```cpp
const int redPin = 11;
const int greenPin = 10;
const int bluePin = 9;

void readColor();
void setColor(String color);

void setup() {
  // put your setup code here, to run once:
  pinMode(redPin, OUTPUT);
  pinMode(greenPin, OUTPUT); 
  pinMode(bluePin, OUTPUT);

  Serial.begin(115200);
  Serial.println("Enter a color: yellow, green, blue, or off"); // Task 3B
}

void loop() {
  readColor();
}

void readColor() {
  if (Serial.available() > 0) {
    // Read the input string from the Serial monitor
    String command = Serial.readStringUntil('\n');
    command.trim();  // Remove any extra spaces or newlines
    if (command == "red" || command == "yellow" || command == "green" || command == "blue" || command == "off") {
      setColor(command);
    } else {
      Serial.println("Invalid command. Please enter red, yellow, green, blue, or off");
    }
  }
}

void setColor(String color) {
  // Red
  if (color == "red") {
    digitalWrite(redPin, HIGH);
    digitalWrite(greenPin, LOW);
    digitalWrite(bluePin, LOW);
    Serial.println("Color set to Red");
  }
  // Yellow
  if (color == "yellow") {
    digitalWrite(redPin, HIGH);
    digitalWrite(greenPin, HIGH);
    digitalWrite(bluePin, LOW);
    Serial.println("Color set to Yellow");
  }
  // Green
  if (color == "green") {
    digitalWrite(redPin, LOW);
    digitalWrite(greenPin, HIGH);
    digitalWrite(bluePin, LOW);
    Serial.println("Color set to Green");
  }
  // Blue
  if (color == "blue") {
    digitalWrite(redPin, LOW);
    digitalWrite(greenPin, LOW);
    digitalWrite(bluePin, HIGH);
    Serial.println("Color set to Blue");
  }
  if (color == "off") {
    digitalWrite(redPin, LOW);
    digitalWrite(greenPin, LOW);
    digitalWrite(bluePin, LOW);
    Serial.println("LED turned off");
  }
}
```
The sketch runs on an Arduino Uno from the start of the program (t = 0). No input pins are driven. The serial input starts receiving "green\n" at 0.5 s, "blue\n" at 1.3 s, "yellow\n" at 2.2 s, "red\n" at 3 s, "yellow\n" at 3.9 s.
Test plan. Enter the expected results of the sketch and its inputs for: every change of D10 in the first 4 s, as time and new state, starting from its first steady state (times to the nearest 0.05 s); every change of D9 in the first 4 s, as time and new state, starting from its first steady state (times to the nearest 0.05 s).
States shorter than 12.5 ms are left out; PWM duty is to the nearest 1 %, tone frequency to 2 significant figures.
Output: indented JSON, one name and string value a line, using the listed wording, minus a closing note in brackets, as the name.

{
  "every change of D10 in the first 4 s, as time and new state, starting from its first steady state": "0 s low; 0.5 s high; 1.3 s low; 2.2 s high; 3 s low; 3.9 s high",
  "every change of D9 in the first 4 s, as time and new state, starting from its first steady state": "0 s low; 1.3 s high; 2.2 s low"
}
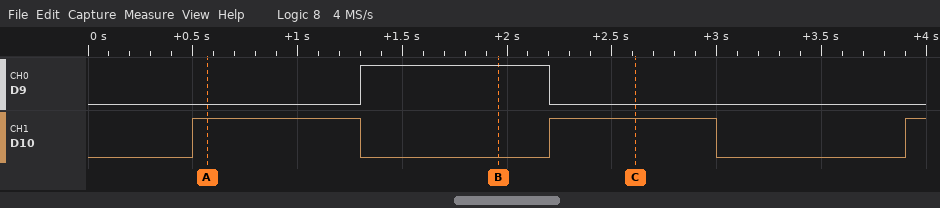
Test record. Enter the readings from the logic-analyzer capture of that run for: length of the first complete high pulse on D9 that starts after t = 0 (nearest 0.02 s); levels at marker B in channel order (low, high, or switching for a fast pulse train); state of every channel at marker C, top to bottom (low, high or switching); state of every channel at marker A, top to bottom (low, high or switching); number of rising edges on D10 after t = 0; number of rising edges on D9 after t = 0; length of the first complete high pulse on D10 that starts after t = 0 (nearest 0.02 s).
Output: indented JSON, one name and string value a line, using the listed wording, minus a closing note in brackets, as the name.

{
  "length of the first complete high pulse on D9 that starts after t = 0": "0.90 s",
  "levels at marker B in channel order": "D9 high, D10 low",
  "state of every channel at marker C, top to bottom": "D9 low, D10 high",
  "state of every channel at marker A, top to bottom": "D9 low, D10 high",
  "number of rising edges on D10 after t = 0": "3",
  "number of rising edges on D9 after t = 0": "1",
  "length of the first complete high pulse on D10 that starts after t = 0": "0.80 s"
}
